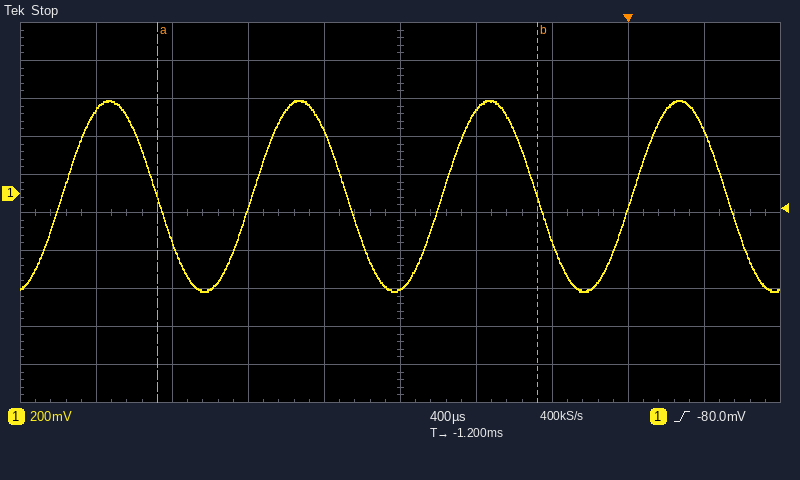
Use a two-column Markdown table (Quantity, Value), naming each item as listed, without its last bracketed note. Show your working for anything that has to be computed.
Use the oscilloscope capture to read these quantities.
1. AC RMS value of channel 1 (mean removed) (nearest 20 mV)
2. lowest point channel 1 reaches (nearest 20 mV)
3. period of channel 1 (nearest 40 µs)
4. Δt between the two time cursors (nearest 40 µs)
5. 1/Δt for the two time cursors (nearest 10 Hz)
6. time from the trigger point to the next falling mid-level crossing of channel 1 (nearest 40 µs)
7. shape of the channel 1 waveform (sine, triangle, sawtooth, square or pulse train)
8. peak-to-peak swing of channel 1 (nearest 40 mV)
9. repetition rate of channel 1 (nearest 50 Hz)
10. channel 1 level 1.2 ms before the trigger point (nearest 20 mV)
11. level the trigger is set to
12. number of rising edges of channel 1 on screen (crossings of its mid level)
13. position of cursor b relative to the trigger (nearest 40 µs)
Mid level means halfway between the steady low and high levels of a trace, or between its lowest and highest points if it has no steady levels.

| Quantity | Value |
|---|---|
| AC RMS value of channel 1 (mean removed) | 1.00 V / (2√2) ≈ 354 mV, so 360 mV to the nearest 20 mV |
| lowest point channel 1 reaches | -520 mV |
| period of channel 1 | 1.00 ms |
| Δt between the two time cursors | 2.00 ms |
| 1/Δt for the two time cursors | 1 / 2.00 ms ≈ 500 Hz |
| time from the trigger point to the next falling mid-level crossing of channel 1 | 520 µs |
| shape of the channel 1 waveform | sine |
| peak-to-peak swing of channel 1 | 1.00 V |
| repetition rate of channel 1 | 1 / 1.00 ms ≈ 1.00 kHz |
| channel 1 level 1.2 ms before the trigger point | -500 mV |
| level the trigger is set to | -80.0 mV |
| number of rising edges of channel 1 on screen | 4 |
| position of cursor b relative to the trigger | -480 µs |
